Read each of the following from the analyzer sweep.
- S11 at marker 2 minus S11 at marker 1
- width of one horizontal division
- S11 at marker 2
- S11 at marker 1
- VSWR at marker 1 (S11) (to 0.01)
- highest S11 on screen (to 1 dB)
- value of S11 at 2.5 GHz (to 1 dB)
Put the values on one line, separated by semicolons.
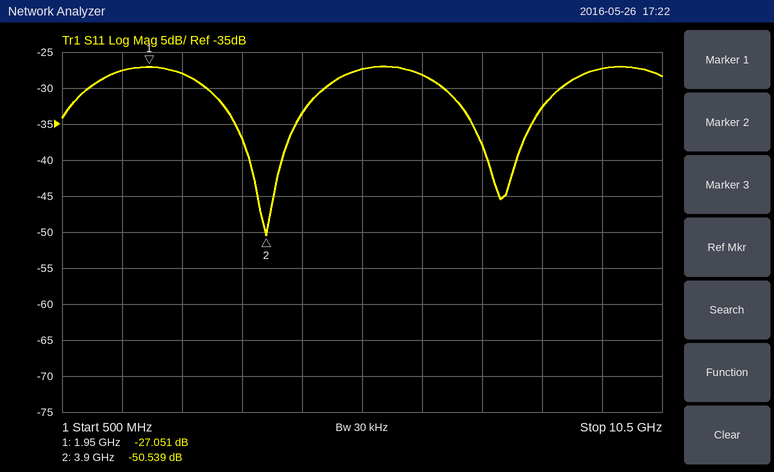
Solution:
-23.488 dB; 1 GHz; -50.539 dB; -27.051 dB; 1.09; -27 dB; -28 dB
